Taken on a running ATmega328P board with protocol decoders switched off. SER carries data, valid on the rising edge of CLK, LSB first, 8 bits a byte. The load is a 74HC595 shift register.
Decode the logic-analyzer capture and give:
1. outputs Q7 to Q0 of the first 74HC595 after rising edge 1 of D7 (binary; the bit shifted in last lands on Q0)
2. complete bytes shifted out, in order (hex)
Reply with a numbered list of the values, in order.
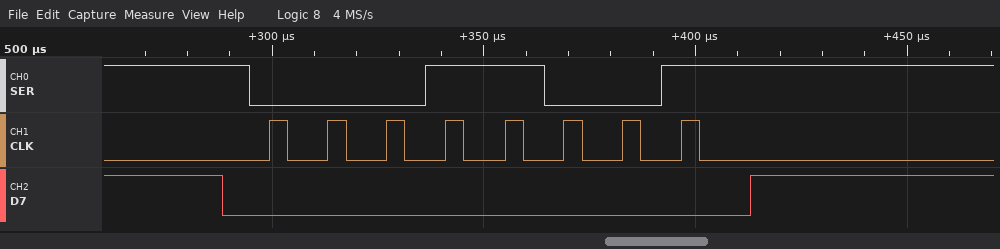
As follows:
1. 00011001
2. 98
